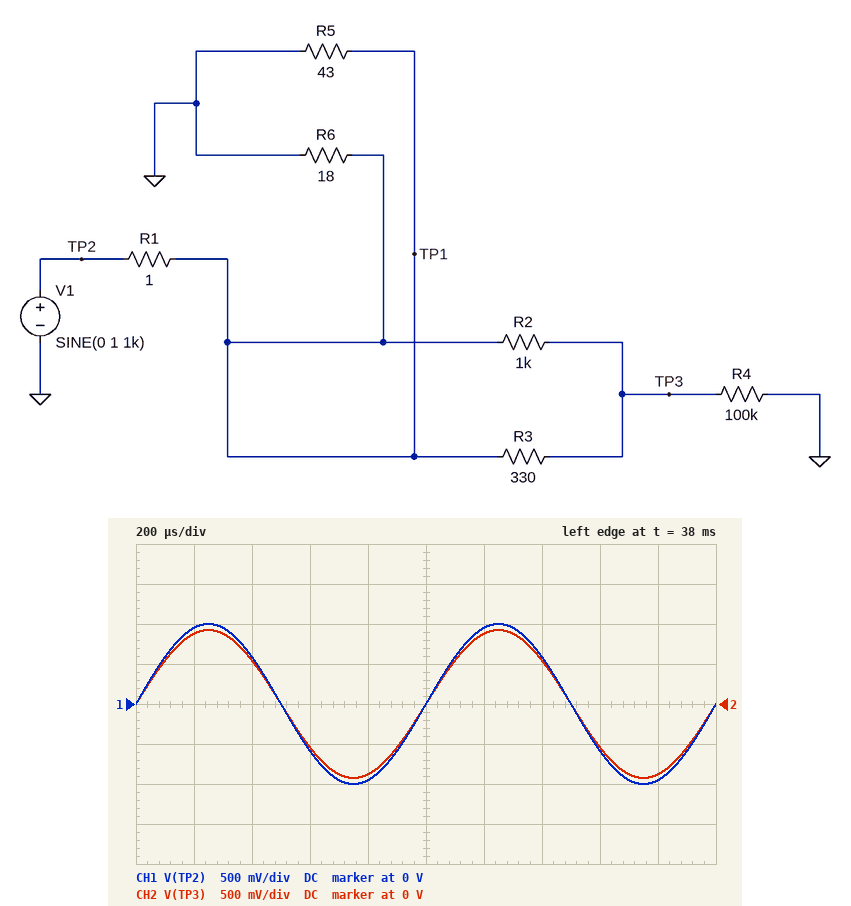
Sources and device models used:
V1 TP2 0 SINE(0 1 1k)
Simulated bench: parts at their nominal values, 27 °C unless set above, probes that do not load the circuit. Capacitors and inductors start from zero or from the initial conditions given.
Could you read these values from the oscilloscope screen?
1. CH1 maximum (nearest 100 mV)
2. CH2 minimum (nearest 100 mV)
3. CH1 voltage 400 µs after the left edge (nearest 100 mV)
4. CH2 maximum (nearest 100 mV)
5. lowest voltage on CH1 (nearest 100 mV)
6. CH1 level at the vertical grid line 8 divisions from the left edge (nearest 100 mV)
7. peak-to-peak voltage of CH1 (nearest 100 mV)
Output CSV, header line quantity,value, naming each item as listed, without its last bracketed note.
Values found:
quantity,value
CH1 maximum,1.0 V
CH2 minimum,-900 mV
CH1 voltage 400 µs after the left edge,600 mV
CH2 maximum,900 mV
lowest voltage on CH1,-1.0 V
CH1 level at the vertical grid line 8 divisions from the left edge,-600 mV
peak-to-peak voltage of CH1,2.0 V
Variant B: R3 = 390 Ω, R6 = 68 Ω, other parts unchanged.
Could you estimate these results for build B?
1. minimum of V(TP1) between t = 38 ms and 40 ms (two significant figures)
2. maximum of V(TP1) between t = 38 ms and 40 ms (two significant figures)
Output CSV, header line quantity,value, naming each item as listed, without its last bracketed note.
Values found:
quantity,value
minimum of V(TP1) between t = 38 ms and 40 ms,-960 mV
maximum of V(TP1) between t = 38 ms and 40 ms,960 mV
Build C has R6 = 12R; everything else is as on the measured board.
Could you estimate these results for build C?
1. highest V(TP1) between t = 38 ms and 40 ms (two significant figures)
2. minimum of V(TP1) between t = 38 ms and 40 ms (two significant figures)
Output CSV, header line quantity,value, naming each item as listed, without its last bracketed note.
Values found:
quantity,value
highest V(TP1) between t = 38 ms and 40 ms,900 mV
minimum of V(TP1) between t = 38 ms and 40 ms,-900 mV
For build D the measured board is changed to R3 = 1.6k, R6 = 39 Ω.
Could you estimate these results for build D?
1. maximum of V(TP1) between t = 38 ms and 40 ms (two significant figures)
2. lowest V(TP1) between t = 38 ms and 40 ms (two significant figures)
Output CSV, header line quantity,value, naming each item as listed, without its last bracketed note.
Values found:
quantity,value
maximum of V(TP1) between t = 38 ms and 40 ms,950 mV
lowest V(TP1) between t = 38 ms and 40 ms,-950 mV
